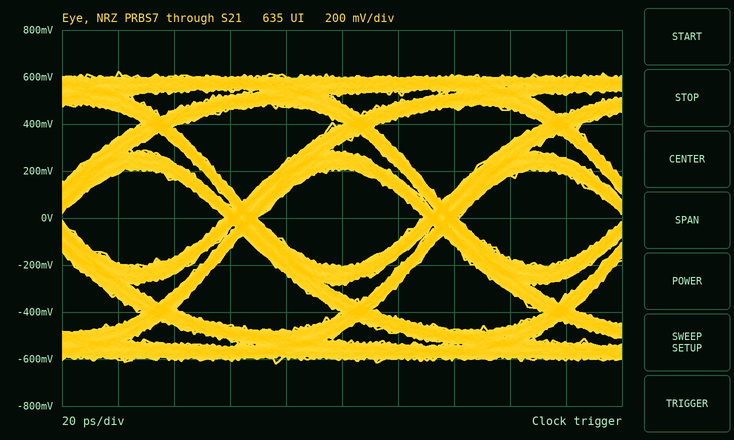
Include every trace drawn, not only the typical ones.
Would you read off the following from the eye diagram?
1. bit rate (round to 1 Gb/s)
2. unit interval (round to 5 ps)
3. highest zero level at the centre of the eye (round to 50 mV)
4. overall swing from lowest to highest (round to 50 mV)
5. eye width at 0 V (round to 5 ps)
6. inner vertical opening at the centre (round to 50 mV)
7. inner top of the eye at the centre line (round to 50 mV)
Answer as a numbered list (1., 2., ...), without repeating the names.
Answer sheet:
1. 14 Gb/s
2. 70 ps
3. -200 mV
4. 1.25 V
5. 60 ps
6. 400 mV
7. 200 mV
